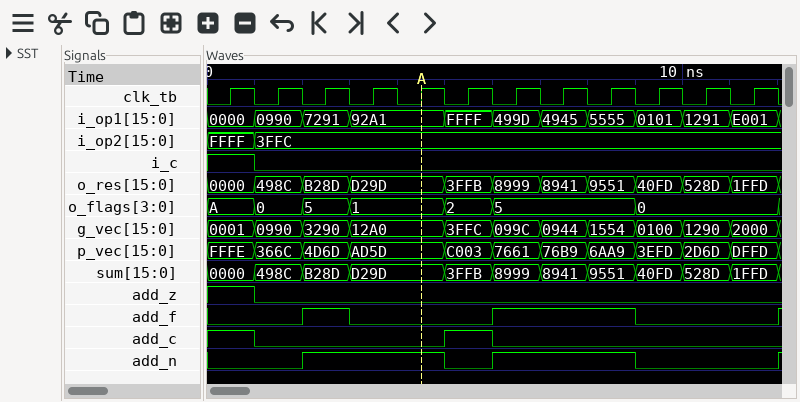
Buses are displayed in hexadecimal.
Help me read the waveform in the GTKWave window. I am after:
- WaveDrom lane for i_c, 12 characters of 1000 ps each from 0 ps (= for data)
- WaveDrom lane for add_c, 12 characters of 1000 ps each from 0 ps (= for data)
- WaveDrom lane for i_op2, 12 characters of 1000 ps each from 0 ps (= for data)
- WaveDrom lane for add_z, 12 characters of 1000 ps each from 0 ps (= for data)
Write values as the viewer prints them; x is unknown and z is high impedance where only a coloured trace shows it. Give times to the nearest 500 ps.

{name: 'i_c', wave: '10..........'}
{name: 'add_c', wave: '10...10.....'}
{name: 'i_op2', wave: '==..........', data: 'FFFF 3FFC'}
{name: 'add_z', wave: '10..........'}
